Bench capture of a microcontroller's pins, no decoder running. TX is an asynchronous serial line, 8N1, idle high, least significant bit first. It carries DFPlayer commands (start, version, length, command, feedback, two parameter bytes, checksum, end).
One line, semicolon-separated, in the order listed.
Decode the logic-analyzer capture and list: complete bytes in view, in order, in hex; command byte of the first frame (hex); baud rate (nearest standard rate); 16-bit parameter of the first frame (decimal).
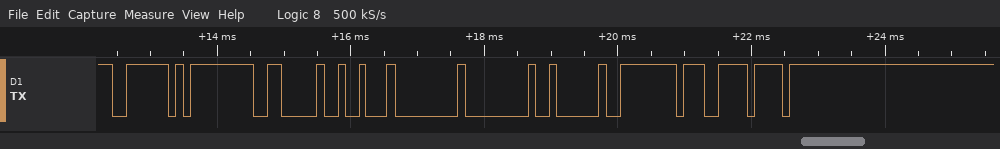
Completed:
0x7E 0xFF 0x06 0x12 0x00 0x00 0x02 0xFE 0xE7 0xEF; 0x12; 9600 baud; 2
